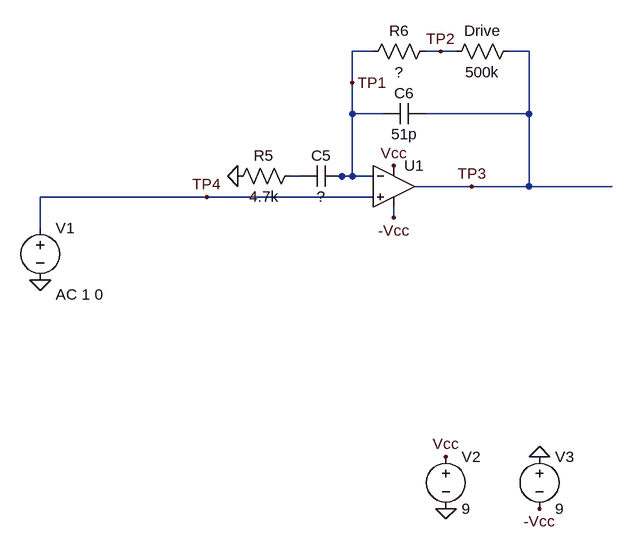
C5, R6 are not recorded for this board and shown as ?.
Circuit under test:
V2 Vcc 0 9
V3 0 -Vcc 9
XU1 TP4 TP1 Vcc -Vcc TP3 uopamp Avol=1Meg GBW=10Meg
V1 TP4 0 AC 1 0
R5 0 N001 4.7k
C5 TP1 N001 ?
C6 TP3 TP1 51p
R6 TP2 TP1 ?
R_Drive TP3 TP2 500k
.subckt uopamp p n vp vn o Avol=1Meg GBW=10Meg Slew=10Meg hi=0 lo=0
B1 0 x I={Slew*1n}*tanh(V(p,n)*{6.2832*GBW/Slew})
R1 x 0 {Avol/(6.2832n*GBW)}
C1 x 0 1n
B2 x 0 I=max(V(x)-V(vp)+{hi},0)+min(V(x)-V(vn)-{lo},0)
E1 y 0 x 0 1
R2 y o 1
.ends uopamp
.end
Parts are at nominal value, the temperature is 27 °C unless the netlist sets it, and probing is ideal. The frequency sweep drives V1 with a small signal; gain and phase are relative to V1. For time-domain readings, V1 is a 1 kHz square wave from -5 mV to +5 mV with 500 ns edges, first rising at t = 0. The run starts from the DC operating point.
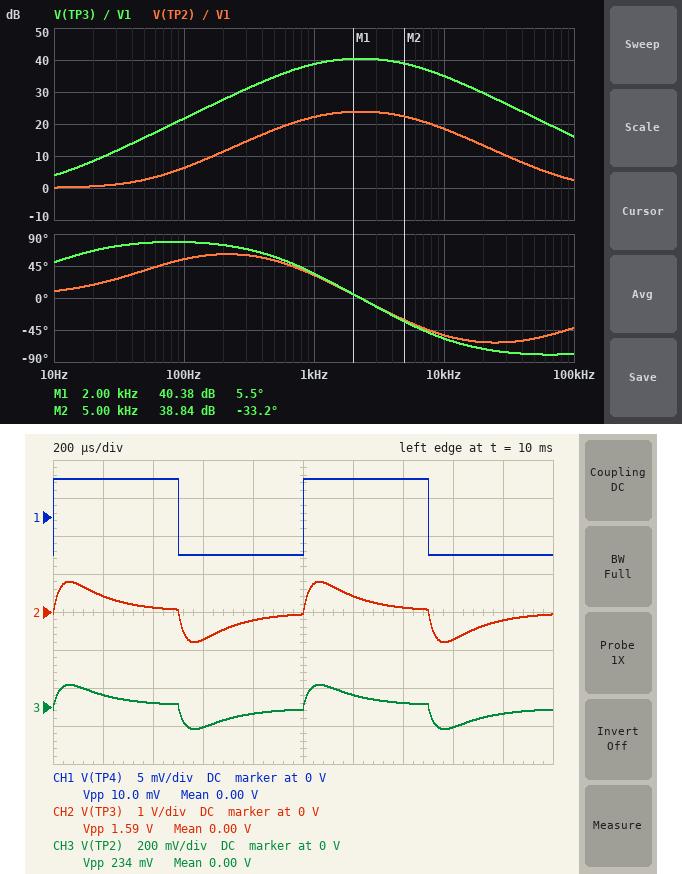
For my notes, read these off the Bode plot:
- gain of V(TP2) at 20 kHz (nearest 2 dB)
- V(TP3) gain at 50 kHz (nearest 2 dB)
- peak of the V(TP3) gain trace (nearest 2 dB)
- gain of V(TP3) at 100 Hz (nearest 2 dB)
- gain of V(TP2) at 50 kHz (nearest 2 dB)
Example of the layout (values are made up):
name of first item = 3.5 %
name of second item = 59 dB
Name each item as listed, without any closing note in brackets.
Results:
gain of V(TP2) at 20 kHz = 14 dB
V(TP3) gain at 50 kHz = 22 dB
peak of the V(TP3) gain trace = 40 dB
gain of V(TP3) at 100 Hz = 22 dB
gain of V(TP2) at 50 kHz = 6 dB
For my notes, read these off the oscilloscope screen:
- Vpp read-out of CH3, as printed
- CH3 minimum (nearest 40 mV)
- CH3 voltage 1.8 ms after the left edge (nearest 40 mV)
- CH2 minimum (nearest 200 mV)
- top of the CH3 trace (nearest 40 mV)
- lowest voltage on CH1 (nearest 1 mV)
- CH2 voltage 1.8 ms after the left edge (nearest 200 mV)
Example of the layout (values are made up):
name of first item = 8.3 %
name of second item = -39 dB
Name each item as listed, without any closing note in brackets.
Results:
Vpp read-out of CH3, as printed = 234 mV
CH3 minimum = -120 mV
CH3 voltage 1.8 ms after the left edge = -40 mV
CH2 minimum = -800 mV
top of the CH3 trace = 120 mV
lowest voltage on CH1 = -5 mV
CH2 voltage 1.8 ms after the left edge = -200 mV
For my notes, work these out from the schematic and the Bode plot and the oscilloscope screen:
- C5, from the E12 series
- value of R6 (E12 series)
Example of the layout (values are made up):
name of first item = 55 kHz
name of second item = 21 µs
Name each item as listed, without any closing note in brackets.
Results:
C5, from the E12 series = 33 nF
value of R6 = 82 kΩ
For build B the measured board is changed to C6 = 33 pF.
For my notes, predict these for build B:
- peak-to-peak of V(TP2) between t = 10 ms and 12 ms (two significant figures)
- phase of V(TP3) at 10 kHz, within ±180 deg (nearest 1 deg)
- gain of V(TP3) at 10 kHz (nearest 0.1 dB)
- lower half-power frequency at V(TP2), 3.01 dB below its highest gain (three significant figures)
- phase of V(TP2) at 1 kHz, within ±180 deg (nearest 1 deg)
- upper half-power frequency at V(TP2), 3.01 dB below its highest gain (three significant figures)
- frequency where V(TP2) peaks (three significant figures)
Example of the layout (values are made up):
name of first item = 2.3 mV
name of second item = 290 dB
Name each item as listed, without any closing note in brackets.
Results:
peak-to-peak of V(TP2) between t = 10 ms and 12 ms = 260 mV
phase of V(TP3) at 10 kHz, within ±180 deg = -47 deg
gain of V(TP3) at 10 kHz = 37.5 dB
lower half-power frequency at V(TP2), 3.01 dB below its highest gain = 829 Hz
phase of V(TP2) at 1 kHz, within ±180 deg = 36 deg
upper half-power frequency at V(TP2), 3.01 dB below its highest gain = 9.30 kHz
frequency where V(TP2) peaks = 2.78 kHz
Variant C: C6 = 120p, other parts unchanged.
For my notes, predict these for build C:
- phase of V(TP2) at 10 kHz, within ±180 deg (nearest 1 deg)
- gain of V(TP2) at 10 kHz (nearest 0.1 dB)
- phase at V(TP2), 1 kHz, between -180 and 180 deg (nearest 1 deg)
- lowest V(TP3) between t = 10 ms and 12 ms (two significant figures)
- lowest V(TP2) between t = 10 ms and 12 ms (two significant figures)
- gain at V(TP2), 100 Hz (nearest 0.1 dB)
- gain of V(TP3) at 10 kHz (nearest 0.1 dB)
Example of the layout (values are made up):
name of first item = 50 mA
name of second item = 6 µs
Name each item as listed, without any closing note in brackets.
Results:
phase of V(TP2) at 10 kHz, within ±180 deg = -59 deg
gain of V(TP2) at 10 kHz = 12.4 dB
phase at V(TP2), 1 kHz, between -180 and 180 deg = 20 deg
lowest V(TP3) between t = 10 ms and 12 ms = -600 mV
lowest V(TP2) between t = 10 ms and 12 ms = -89 mV
gain at V(TP2), 100 Hz = 6.4 dB
gain of V(TP3) at 10 kHz = 28.6 dB
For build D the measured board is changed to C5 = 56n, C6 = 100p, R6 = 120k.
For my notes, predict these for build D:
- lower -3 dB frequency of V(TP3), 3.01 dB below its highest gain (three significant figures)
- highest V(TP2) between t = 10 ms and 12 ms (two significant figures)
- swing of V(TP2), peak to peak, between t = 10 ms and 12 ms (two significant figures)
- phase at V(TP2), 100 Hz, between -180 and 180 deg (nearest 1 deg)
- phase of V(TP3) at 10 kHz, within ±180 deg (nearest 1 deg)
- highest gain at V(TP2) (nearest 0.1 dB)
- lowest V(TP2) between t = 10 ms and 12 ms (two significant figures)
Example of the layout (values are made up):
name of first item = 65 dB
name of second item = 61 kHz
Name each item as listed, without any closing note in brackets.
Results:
lower -3 dB frequency of V(TP3), 3.01 dB below its highest gain = 429 Hz
highest V(TP2) between t = 10 ms and 12 ms = 140 mV
swing of V(TP2), peak to peak, between t = 10 ms and 12 ms = 280 mV
phase at V(TP2), 100 Hz, between -180 and 180 deg = 66 deg
phase of V(TP3) at 10 kHz, within ±180 deg = -71 deg
highest gain at V(TP2) = 26.7 dB
lowest V(TP2) between t = 10 ms and 12 ms = -140 mV
